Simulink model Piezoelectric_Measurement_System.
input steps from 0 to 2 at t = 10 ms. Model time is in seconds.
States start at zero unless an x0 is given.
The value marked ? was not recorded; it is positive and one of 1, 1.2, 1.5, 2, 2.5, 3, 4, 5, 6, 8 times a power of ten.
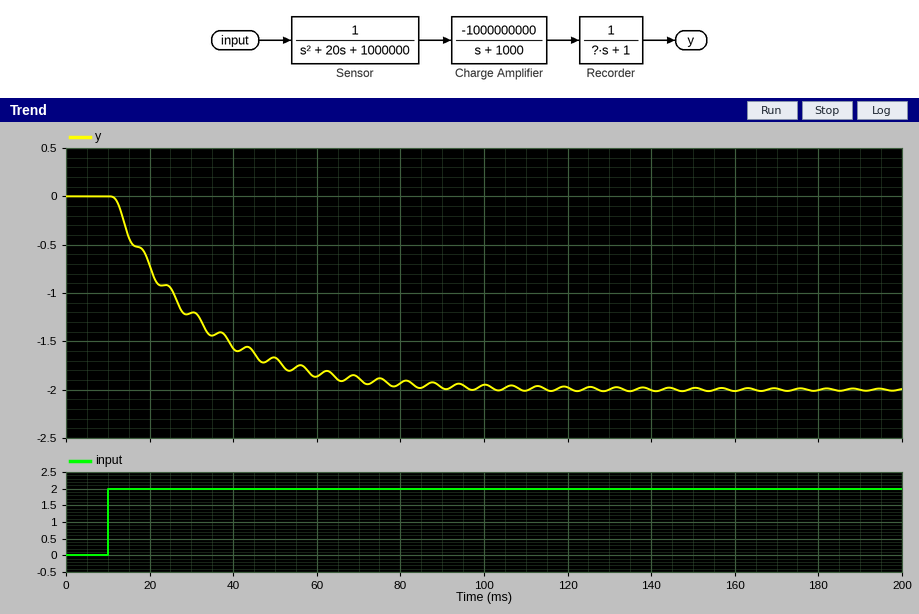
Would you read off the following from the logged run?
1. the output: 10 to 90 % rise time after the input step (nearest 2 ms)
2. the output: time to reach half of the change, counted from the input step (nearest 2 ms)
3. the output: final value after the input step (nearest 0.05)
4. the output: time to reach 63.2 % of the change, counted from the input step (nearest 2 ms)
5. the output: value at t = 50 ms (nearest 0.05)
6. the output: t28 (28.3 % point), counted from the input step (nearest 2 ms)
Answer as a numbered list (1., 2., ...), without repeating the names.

1. 40 ms
2. 16 ms
3. -2.00
4. 22 ms
5. -1.65
6. 8 ms
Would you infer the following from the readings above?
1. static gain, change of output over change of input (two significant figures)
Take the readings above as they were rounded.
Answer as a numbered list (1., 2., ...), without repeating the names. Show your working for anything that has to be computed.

1. (-2 - 0) / (2 - 0) = -1.0
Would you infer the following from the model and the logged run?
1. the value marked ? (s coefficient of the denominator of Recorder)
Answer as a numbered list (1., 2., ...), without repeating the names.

1. 0.02
